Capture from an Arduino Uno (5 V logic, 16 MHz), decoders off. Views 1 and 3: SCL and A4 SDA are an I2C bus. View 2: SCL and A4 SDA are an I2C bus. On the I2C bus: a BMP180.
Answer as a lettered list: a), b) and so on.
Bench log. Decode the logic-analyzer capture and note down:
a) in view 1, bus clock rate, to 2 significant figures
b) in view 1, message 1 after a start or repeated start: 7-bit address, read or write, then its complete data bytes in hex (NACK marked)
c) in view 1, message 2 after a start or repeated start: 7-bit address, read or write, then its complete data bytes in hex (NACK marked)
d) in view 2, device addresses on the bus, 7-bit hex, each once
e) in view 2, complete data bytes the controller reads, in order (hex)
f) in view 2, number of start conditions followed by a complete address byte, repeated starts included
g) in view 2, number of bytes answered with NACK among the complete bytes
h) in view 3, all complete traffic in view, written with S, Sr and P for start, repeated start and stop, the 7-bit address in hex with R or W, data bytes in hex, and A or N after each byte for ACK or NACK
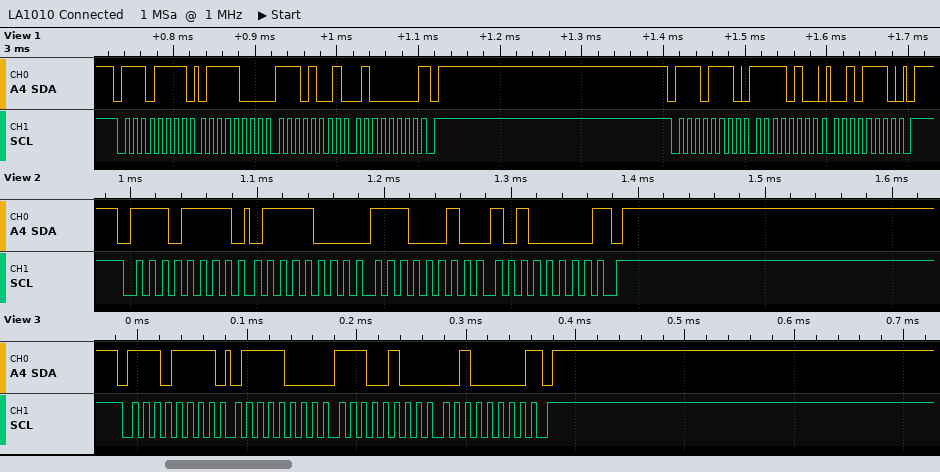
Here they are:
a) 100 kHz
b) 0x77 read: 78 E9 40 NACK
c) 0x77 write: F4 2E
d) 0x77
e) 78 E2 A0
f) 1
g) 1
h) S 77R A 78 A E4 A 20 N P
